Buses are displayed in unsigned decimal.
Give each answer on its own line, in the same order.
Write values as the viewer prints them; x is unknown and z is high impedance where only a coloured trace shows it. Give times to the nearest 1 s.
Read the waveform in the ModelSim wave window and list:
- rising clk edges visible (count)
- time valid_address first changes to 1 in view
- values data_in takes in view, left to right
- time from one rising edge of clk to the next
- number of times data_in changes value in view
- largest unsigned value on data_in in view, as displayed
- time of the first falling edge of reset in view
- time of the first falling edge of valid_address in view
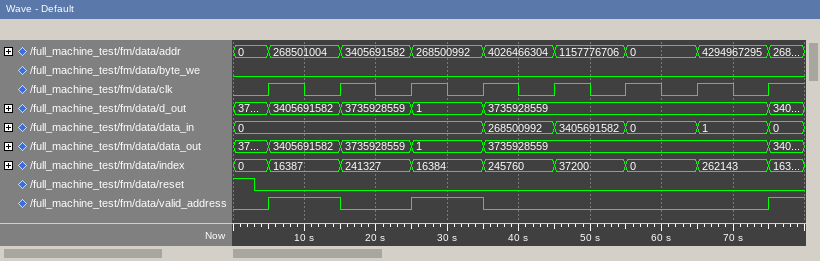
8
5 s
0, 268500992, 3405691582, 0, 1, 0
10 s
5
3405691582
3 s
15 s
